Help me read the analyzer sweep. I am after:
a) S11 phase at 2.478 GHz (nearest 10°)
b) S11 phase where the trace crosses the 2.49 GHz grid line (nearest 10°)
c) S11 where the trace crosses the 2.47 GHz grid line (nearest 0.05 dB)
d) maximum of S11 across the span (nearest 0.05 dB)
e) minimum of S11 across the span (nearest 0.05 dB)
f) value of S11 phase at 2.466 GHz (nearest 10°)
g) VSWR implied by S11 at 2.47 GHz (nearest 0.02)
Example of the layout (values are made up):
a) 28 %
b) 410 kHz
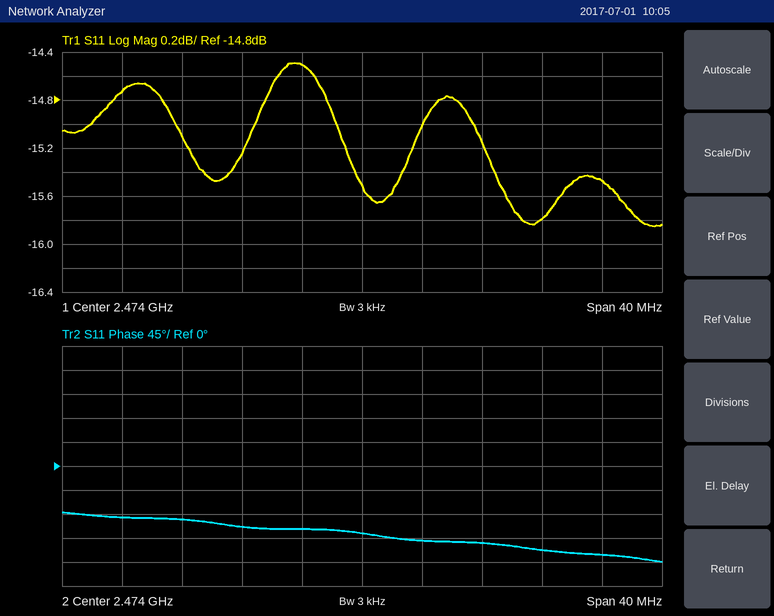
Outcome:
a) -140°
b) -170°
c) -14.50 dB
d) -14.50 dB
e) -15.85 dB
f) -110°
g) 1.46
